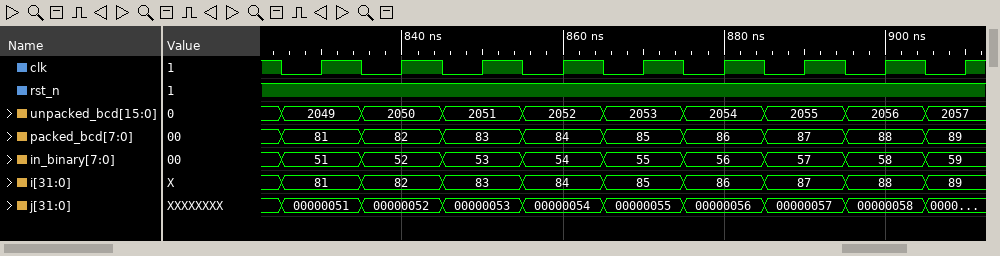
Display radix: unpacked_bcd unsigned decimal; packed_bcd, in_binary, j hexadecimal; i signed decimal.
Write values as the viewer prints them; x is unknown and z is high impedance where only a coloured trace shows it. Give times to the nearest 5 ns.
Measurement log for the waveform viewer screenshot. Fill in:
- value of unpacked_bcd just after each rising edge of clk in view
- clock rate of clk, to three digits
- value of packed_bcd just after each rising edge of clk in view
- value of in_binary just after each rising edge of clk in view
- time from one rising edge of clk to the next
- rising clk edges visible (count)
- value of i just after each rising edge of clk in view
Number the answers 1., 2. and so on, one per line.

1. 2049, 2050, 2051, 2052, 2053, 2054, 2055, 2056, 2057
2. 100 MHz
3. 81, 82, 83, 84, 85, 86, 87, 88, 89
4. 51, 52, 53, 54, 55, 56, 57, 58, 59
5. 10 ns
6. 9
7. 81, 82, 83, 84, 85, 86, 87, 88, 89
